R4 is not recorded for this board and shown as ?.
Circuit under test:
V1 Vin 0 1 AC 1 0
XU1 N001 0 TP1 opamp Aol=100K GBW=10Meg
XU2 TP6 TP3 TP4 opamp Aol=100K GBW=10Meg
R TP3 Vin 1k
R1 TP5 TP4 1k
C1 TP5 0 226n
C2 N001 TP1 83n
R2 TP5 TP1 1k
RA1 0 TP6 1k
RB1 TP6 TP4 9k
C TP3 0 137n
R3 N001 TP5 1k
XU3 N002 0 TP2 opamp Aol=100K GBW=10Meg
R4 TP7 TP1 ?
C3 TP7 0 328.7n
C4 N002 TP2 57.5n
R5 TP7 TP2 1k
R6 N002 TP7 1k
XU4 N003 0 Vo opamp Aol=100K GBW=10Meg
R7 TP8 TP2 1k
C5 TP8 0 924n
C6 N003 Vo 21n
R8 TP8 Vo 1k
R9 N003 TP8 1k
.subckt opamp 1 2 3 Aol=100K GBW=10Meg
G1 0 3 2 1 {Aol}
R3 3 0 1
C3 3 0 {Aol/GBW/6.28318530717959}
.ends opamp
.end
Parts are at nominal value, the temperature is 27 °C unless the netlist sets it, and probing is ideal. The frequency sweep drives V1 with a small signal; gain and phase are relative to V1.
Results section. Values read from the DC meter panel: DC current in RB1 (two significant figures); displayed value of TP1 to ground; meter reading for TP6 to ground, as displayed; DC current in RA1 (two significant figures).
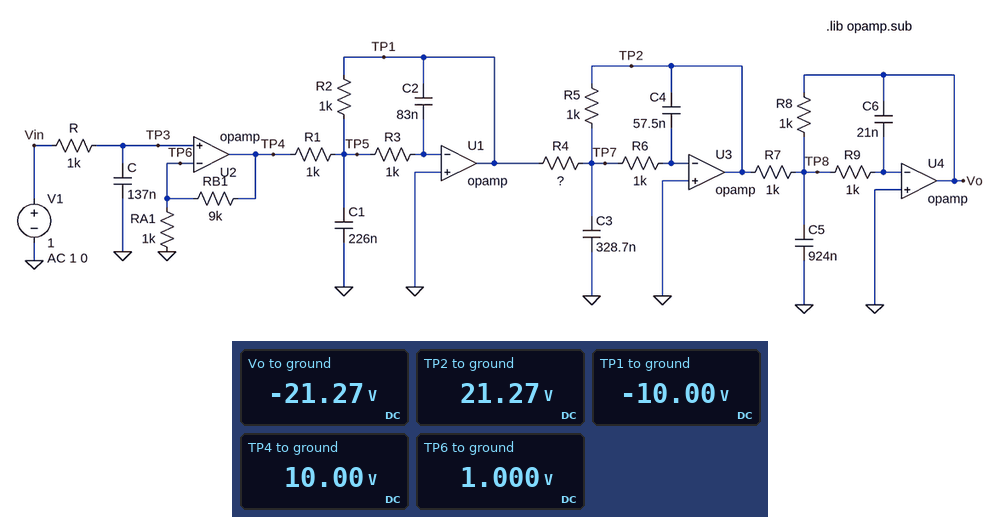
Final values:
1.0 mA
-10.00 V
1.000 V
1.0 mA
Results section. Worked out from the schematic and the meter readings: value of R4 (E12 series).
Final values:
470 Ω
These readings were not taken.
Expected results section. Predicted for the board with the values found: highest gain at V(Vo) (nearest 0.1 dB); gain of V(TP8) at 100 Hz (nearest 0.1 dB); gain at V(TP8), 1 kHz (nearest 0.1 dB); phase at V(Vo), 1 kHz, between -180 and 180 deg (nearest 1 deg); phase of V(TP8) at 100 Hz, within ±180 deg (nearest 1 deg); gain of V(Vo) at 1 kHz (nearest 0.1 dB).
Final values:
26.6 dB
-11.1 dB
5.7 dB
-81 deg
65 deg
23.3 dB
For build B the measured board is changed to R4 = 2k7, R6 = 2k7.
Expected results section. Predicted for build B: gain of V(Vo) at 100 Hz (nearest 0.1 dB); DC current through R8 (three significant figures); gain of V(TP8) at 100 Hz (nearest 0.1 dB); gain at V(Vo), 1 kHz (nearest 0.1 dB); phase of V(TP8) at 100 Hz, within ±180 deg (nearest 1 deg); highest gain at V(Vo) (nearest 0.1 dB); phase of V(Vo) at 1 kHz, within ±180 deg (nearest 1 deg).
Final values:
11.4 dB
3.70 mA
-26.2 dB
5.8 dB
64 deg
11.6 dB
-122 deg
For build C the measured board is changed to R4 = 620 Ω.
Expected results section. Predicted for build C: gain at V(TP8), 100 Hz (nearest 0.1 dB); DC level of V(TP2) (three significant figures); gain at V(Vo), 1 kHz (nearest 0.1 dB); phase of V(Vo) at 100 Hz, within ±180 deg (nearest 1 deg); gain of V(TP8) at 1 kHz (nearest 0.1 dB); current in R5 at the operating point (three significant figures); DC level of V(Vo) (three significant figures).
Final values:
-13.5 dB
16.1 V
22.0 dB
156 deg
4.4 dB
16.1 mA
-16.1 V
